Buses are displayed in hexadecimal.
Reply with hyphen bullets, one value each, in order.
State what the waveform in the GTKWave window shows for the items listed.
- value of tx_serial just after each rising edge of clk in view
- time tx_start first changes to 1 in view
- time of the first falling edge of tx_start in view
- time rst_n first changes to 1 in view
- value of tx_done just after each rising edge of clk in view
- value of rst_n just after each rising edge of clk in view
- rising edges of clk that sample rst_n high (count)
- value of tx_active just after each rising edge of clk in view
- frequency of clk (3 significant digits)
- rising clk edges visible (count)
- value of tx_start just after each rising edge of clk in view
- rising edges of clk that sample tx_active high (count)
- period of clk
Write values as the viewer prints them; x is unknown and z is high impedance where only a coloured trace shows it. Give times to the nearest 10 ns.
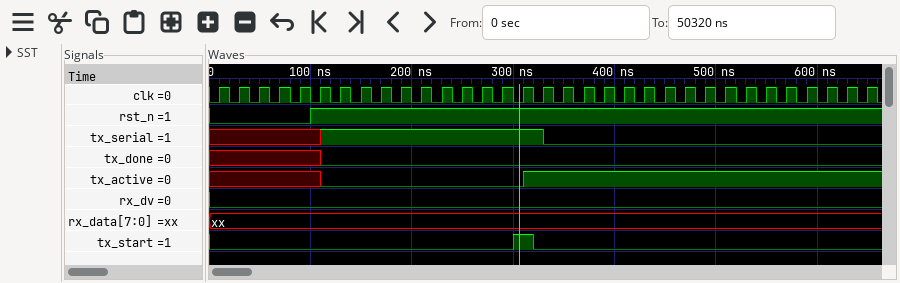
- x x x x x 1 1 1 1 1 1 1 1 1 1 1 0 0 0 0 0 0 0 0 0 0 0 0 0 0 0 0 0
- 300 ns
- 320 ns
- 100 ns
- x x x x x 0 0 0 0 0 0 0 0 0 0 0 0 0 0 0 0 0 0 0 0 0 0 0 0 0 0 0 0
- 0 0 0 0 0 1 1 1 1 1 1 1 1 1 1 1 1 1 1 1 1 1 1 1 1 1 1 1 1 1 1 1 1
- 28
- x x x x x 0 0 0 0 0 0 0 0 0 0 1 1 1 1 1 1 1 1 1 1 1 1 1 1 1 1 1 1
- 50.0 MHz
- 33
- 0 0 0 0 0 0 0 0 0 0 0 0 0 0 0 1 0 0 0 0 0 0 0 0 0 0 0 0 0 0 0 0 0
- 17
- 20 ns
